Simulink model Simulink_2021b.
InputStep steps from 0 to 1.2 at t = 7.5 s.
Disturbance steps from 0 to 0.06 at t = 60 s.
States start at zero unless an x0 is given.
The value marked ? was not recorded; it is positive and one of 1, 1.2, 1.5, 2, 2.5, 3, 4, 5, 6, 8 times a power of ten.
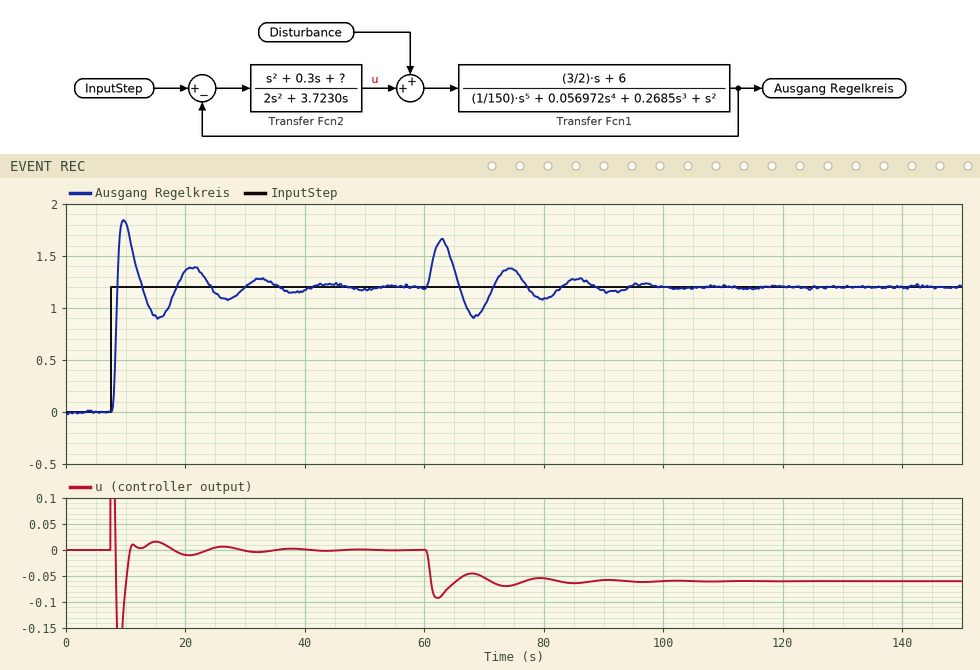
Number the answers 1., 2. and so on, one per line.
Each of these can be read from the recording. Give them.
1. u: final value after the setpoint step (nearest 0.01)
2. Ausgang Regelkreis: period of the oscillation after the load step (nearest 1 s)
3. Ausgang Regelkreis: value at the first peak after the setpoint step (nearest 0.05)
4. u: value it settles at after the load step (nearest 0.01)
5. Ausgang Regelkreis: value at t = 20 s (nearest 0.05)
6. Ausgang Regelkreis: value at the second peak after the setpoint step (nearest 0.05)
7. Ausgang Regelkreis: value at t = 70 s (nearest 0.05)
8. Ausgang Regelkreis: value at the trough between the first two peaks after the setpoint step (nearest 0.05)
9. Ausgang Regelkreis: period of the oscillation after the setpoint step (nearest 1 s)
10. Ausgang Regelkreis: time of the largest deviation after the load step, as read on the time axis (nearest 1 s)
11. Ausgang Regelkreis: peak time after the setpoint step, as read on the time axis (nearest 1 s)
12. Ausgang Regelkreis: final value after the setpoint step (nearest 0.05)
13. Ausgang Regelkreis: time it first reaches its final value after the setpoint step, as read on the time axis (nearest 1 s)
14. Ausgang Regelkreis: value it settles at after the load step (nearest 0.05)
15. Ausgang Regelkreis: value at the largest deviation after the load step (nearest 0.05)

1. 0.00
2. 11 s
3. 1.85
4. -0.06
5. 1.35
6. 1.40
7. 1.00
8. 0.90
9. 11 s
10. 63 s
11. 10 s
12. 1.20
13. 9 s
14. 1.20
15. 1.65
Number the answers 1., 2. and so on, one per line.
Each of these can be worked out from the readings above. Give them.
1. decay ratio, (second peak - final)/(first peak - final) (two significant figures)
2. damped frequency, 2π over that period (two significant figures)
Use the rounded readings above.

1. 0.31
2. 0.57 rad/s
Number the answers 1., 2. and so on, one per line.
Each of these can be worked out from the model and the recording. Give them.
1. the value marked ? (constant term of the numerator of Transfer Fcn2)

1. 0.25
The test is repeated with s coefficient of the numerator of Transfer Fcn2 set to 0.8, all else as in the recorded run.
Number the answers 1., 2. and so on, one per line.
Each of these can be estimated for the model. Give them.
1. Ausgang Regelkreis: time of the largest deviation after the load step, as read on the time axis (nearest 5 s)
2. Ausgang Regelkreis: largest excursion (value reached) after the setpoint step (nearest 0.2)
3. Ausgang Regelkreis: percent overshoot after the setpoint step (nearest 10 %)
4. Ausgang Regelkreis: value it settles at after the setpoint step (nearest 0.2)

1. 60 s
2. 2.2
3. 90 %
4. 1.2
